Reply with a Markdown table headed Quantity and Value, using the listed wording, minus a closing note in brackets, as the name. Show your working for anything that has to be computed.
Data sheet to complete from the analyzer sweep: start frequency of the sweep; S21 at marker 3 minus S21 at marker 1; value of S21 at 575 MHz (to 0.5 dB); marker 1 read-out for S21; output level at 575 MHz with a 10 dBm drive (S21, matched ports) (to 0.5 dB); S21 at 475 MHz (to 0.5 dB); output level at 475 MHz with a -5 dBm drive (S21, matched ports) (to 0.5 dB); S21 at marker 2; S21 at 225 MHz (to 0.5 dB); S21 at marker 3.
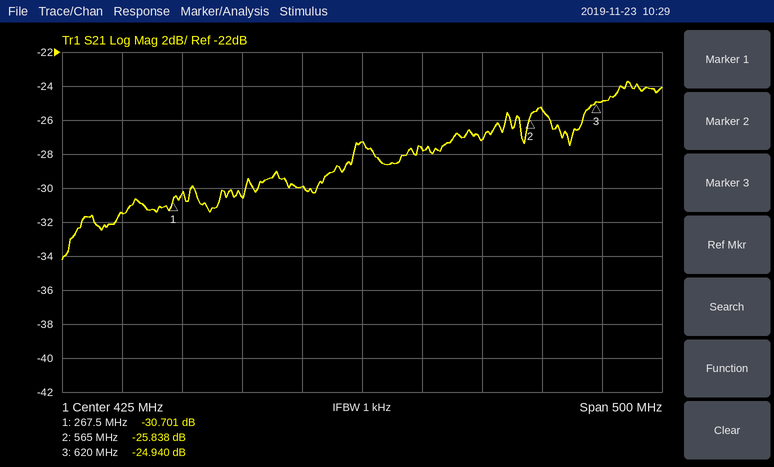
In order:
| Quantity | Value |
|---|---|
| start frequency of the sweep | 175 MHz |
| S21 at marker 3 minus S21 at marker 1 | -24.94 − (-30.701) = 5.761 dB |
| value of S21 at 575 MHz | -25.5 dB |
| marker 1 read-out for S21 | -30.701 dB |
| output level at 575 MHz with a 10 dBm drive (S21, matched ports) | 10 dBm + (-25.5 dB) = -15.5 dBm |
| S21 at 475 MHz | -27.5 dB |
| output level at 475 MHz with a -5 dBm drive (S21, matched ports) | -5 dBm + (-27.5 dB) = -32.5 dBm |
| S21 at marker 2 | -25.838 dB |
| S21 at 225 MHz | -31.5 dB |
| S21 at marker 3 | -24.940 dB |
